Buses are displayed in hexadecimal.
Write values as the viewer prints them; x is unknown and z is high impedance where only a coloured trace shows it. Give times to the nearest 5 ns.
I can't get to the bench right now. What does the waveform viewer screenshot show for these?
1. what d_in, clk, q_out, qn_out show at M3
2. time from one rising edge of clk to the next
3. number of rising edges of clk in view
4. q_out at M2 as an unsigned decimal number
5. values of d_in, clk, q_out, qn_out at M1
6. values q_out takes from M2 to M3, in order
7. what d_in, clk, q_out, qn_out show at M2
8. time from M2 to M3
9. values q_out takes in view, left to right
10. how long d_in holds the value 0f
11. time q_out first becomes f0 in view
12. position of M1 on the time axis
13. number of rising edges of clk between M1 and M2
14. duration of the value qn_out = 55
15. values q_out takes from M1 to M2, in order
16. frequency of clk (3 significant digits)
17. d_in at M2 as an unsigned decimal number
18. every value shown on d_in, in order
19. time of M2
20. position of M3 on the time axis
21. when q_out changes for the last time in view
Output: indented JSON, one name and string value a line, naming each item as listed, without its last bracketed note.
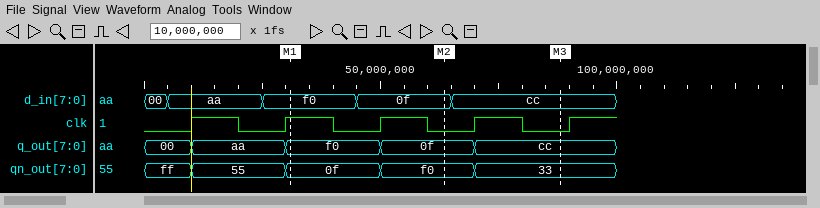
{
  "what d_in, clk, q_out, qn_out show at M3": "d_in=cc, clk=0, q_out=cc, qn_out=33",
  "time from one rising edge of clk to the next": "20 ns",
  "number of rising edges of clk in view": "5",
  "q_out at M2 as an unsigned decimal number": "15",
  "values of d_in, clk, q_out, qn_out at M1": "d_in=f0, clk=1, q_out=f0, qn_out=0f",
  "values q_out takes from M2 to M3, in order": "0f, cc",
  "what d_in, clk, q_out, qn_out show at M2": "d_in=0f, clk=0, q_out=0f, qn_out=f0",
  "time from M2 to M3": "25 ns",
  "values q_out takes in view, left to right": "00, aa, f0, 0f, cc",
  "how long d_in holds the value 0f": "20 ns",
  "time q_out first becomes f0 in view": "30 ns",
  "position of M1 on the time axis": "30 ns",
  "number of rising edges of clk between M1 and M2": "1",
  "duration of the value qn_out = 55": "20 ns",
  "values q_out takes from M1 to M2, in order": "f0, 0f",
  "frequency of clk": "50.0 MHz",
  "d_in at M2 as an unsigned decimal number": "15",
  "every value shown on d_in, in order": "00, aa, f0, 0f, cc",
  "time of M2": "65 ns",
  "position of M3 on the time axis": "90 ns",
  "when q_out changes for the last time in view": "70 ns"
}
